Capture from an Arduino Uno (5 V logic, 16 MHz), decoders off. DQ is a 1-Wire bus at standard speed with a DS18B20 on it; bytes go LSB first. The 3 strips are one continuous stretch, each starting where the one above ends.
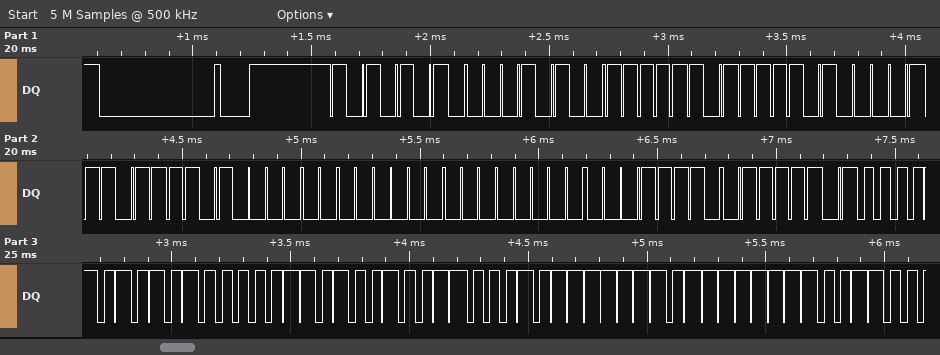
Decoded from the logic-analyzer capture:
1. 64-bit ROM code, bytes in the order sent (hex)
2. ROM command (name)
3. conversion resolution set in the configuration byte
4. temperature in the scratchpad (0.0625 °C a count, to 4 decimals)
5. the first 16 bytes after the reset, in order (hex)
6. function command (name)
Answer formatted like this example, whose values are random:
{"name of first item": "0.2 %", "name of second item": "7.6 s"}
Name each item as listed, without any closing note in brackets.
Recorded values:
{"64-bit ROM code, bytes in the order sent": "28 BF 2F DC 0B 00 00 78", "ROM command": "Match ROM", "conversion resolution set in the configuration byte": "12 bits", "temperature in the scratchpad": "85.0000 °C", "the first 16 bytes after the reset, in order": "55 28 BF 2F DC 0B 00 00 78 BE 50 05 4B 46 7F FF", "function command": "Read Scratchpad"}
